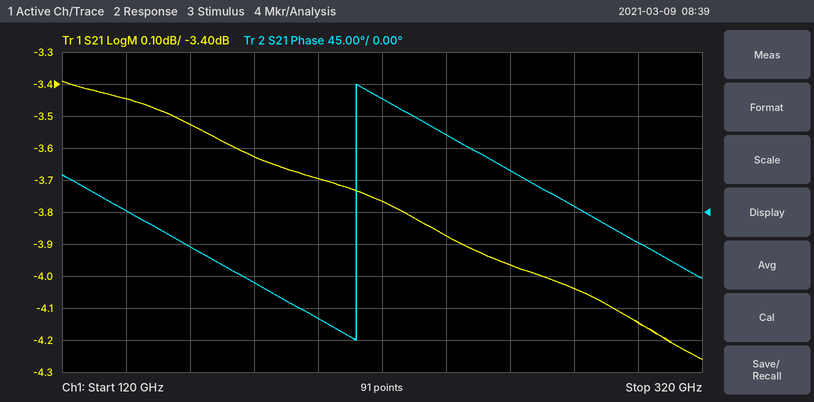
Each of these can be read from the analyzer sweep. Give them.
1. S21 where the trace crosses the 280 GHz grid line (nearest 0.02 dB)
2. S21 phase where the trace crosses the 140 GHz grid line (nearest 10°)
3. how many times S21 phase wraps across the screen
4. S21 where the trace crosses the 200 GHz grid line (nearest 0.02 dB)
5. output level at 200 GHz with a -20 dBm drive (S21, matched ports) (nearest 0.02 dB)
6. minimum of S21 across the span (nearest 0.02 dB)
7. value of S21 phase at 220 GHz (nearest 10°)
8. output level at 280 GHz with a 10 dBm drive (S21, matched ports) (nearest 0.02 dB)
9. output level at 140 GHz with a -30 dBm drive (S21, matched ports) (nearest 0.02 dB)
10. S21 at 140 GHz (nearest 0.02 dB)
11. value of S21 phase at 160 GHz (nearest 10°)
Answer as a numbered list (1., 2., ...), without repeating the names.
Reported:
1. -4.04 dB
2. 0°
3. 1
4. -3.70 dB
5. -23.70 dBm
6. -4.26 dB
7. 160°
8. 5.96 dBm
9. -33.44 dBm
10. -3.44 dB
11. -50°
